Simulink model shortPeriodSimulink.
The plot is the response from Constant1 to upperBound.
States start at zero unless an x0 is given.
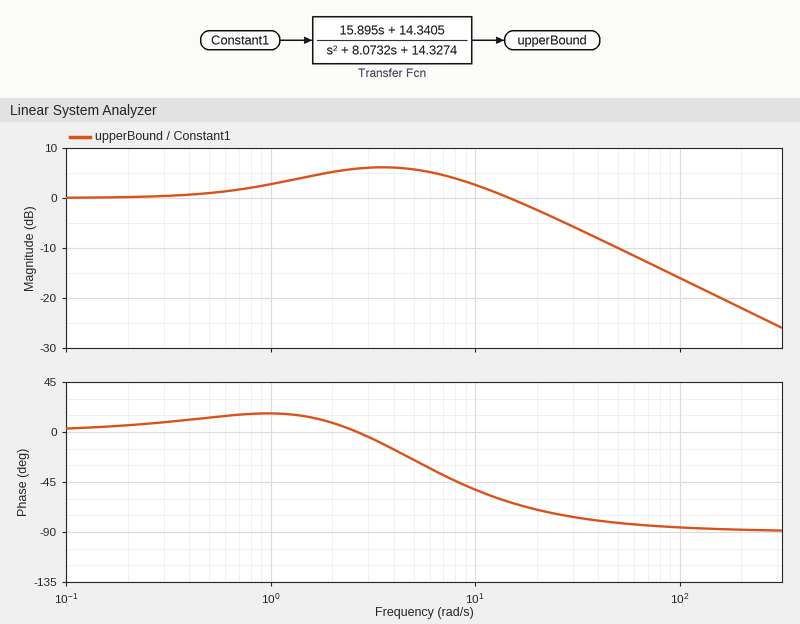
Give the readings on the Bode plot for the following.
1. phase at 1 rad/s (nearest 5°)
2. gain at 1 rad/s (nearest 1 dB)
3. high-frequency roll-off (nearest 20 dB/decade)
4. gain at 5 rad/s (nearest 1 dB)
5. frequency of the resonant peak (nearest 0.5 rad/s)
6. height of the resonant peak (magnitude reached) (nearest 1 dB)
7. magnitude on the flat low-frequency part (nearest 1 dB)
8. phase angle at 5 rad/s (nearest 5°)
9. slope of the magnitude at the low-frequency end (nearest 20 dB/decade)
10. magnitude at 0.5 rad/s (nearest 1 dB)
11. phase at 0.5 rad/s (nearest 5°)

15°
3 dB
-20 dB/decade
6 dB
3.5 rad/s
6 dB
0 dB
-25°
0 dB/decade
1 dB
15°
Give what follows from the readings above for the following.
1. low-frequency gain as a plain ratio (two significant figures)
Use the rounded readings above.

1.0
